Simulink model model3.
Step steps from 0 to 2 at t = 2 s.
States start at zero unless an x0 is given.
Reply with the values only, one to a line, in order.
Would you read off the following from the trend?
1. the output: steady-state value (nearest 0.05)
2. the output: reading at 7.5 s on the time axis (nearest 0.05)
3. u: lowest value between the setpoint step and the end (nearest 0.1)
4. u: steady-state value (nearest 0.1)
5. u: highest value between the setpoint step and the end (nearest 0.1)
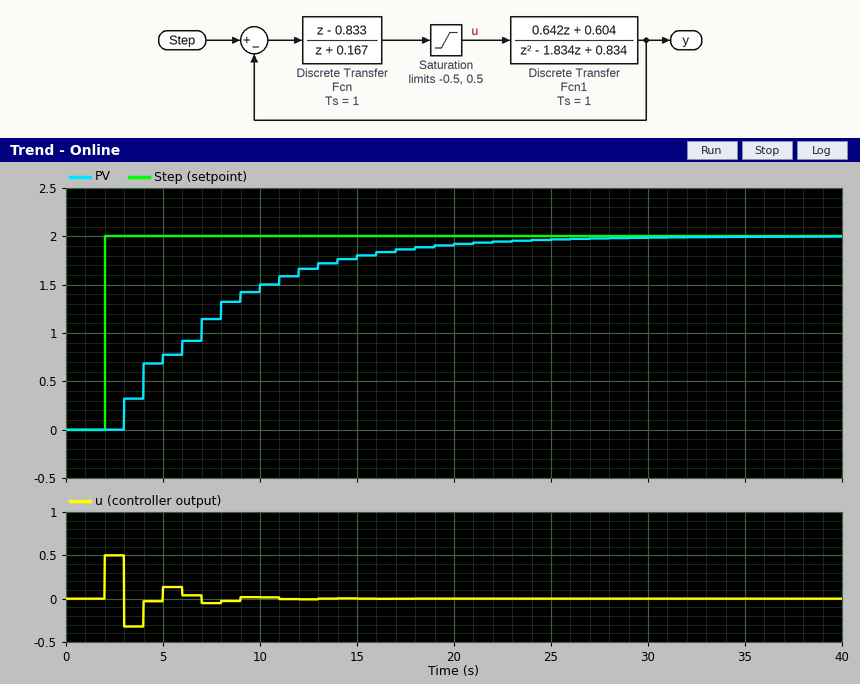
2.00
1.15
-0.3
0.0
0.5
